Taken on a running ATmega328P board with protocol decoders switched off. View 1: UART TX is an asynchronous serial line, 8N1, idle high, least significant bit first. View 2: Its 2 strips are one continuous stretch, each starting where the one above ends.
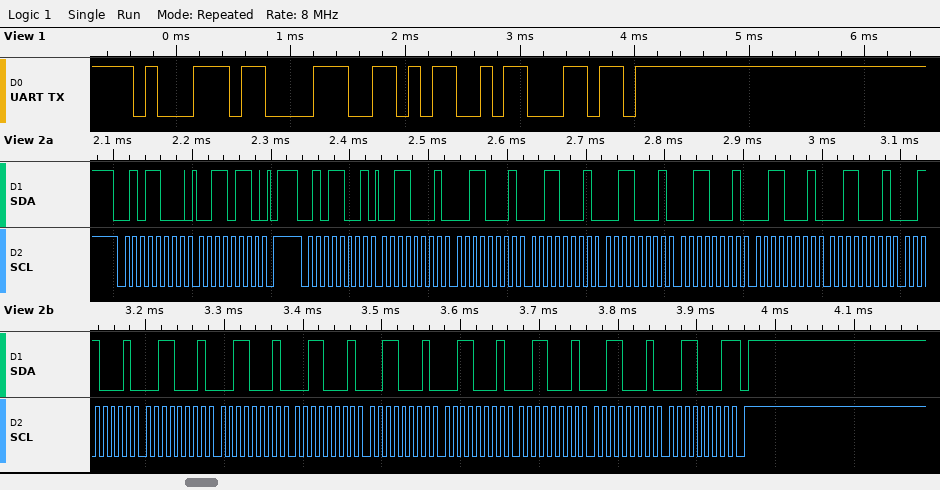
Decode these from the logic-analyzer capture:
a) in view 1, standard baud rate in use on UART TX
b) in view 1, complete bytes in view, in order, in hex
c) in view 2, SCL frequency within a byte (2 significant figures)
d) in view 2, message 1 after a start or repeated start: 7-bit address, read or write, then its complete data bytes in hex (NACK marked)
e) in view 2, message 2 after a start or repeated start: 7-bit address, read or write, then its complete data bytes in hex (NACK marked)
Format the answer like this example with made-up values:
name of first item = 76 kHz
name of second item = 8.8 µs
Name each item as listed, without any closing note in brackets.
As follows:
in view 1, standard baud rate in use on UART TX = 9600 baud
in view 1, complete bytes in view, in order, in hex = 71 38 4D 6C
in view 2, SCL frequency within a byte = 100 kHz
in view 2, message 1 after a start or repeated start: 7-bit address, read or write, then its complete data bytes in hex = 0x2C write: 36
in view 2, message 2 after a start or repeated start: 7-bit address, read or write, then its complete data bytes in hex = 0x2C read: 31 31 31 31 31 31 31 31 31 31 31 31 31 31 31 31 NACK
